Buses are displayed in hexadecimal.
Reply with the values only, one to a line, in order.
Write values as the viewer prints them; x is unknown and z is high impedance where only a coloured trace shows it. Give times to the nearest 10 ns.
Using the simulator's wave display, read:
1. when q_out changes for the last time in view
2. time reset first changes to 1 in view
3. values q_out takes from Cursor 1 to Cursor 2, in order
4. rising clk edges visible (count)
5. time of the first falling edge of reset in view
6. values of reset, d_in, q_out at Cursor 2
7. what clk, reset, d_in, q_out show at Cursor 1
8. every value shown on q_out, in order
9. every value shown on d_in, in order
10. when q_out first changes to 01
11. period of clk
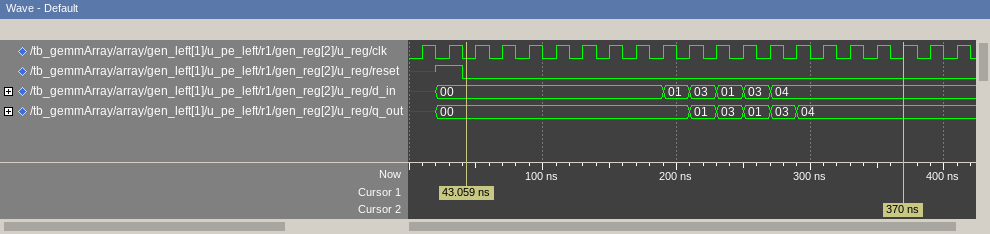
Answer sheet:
290 ns
20 ns
00, 01, 03, 01, 03, 04
21
40 ns
reset=0, d_in=04, q_out=04
clk=0, reset=0, d_in=00, q_out=00
x, 00, 01, 03, 01, 03, 04
x, 00, 01, 03, 01, 03, 04
210 ns
20 ns
